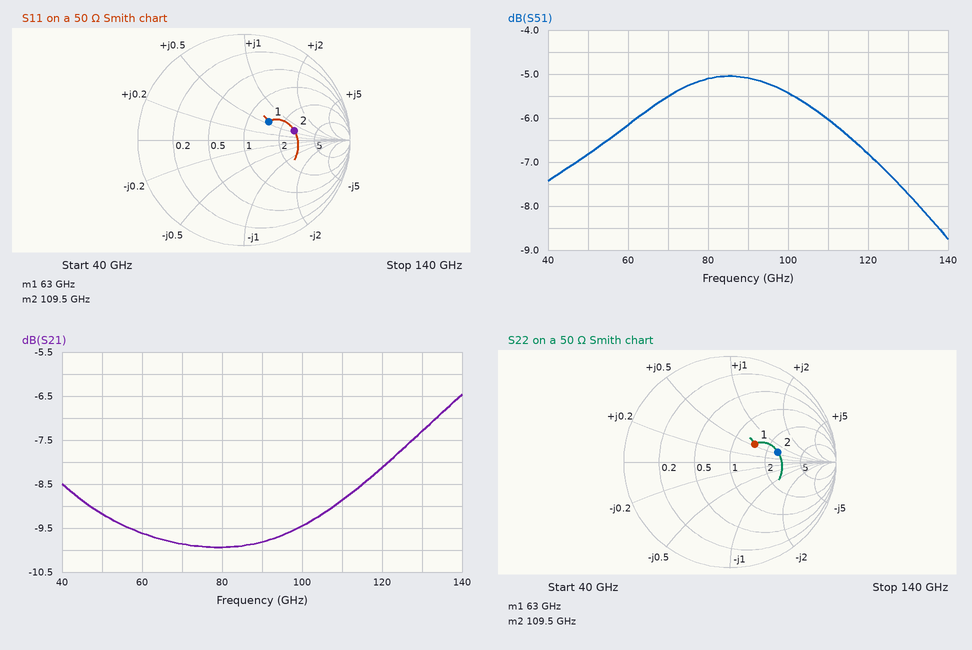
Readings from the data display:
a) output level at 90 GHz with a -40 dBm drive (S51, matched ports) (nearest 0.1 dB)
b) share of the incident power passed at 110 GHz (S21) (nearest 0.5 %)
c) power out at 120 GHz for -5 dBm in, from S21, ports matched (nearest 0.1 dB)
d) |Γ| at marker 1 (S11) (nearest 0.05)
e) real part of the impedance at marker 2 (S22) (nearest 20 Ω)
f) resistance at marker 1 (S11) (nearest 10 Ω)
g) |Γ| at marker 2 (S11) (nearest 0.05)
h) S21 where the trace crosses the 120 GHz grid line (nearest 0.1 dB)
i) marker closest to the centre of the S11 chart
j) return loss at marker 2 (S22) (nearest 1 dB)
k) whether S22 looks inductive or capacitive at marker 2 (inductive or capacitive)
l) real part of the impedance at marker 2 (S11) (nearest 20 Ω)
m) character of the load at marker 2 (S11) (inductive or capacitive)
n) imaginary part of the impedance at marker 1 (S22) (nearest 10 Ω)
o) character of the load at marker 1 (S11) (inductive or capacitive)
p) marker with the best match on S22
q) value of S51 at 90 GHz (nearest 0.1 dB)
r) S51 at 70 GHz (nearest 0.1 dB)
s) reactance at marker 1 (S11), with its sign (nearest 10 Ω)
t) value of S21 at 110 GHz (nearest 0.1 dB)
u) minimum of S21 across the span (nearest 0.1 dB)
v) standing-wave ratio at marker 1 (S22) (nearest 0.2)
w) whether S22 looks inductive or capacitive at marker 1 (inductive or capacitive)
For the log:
-45.1 dBm
13.0 %
-13.1 dBm
0.30
120 Ω
70 Ω
0.50
-8.1 dB
marker 1
7 dB
inductive
140 Ω
inductive
+30 Ω
inductive
marker 1
-5.1 dB
-5.5 dB
+30 Ω
-8.9 dB
-9.9 dB
1.8
inductive
